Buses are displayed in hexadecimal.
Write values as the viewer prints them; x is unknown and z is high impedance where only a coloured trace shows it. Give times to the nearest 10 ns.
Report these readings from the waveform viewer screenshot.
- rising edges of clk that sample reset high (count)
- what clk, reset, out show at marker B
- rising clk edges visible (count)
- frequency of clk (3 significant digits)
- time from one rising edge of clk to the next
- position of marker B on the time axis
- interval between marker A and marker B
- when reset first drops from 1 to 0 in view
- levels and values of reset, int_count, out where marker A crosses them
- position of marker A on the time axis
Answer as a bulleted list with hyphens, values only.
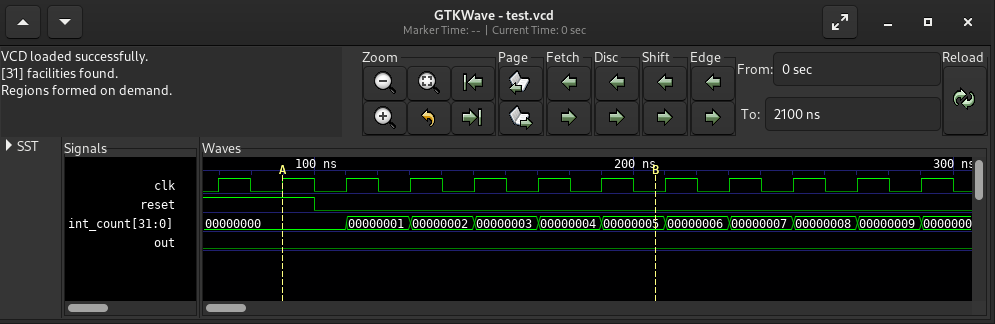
- 2
- clk=0, reset=0, out=0
- 12
- 50.0 MHz
- 20 ns
- 210 ns
- 120 ns
- 100 ns
- reset=1, int_count=00000000, out=0
- 90 ns
